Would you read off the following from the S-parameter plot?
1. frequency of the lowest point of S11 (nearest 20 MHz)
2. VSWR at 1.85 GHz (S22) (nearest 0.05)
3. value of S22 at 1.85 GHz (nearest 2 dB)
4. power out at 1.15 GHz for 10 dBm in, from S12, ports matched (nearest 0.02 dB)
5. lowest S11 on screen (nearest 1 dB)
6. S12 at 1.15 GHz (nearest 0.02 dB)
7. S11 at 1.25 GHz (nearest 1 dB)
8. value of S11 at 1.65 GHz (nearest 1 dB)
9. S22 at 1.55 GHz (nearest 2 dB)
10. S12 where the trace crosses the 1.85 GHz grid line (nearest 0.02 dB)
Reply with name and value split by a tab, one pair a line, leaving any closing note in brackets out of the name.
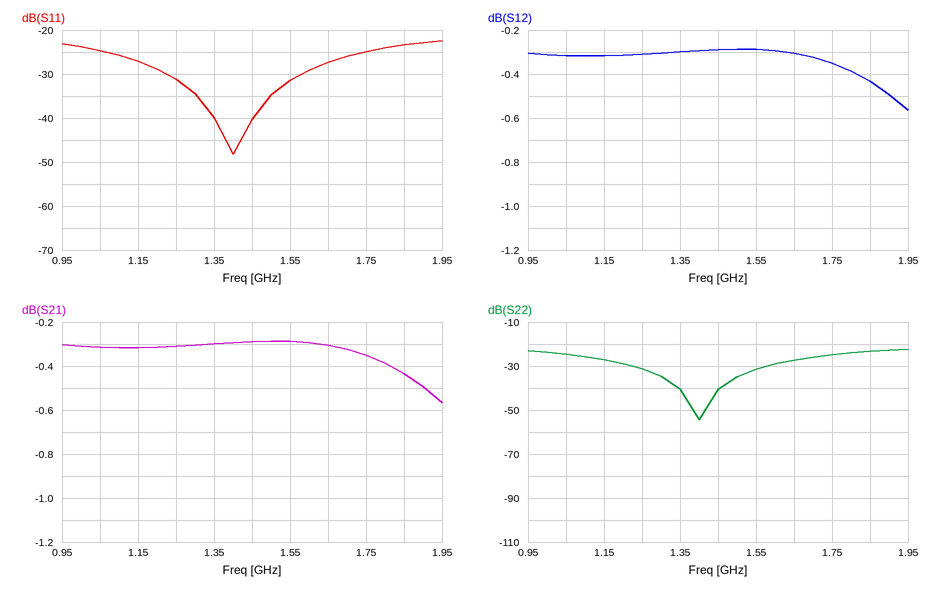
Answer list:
frequency of the lowest point of S11	1.40 GHz
VSWR at 1.85 GHz (S22)	1.15
value of S22 at 1.85 GHz	-24 dB
power out at 1.15 GHz for 10 dBm in, from S12, ports matched	9.68 dBm
lowest S11 on screen	-48 dB
S12 at 1.15 GHz	-0.32 dB
S11 at 1.25 GHz	-31 dB
value of S11 at 1.65 GHz	-27 dB
S22 at 1.55 GHz	-32 dB
S12 where the trace crosses the 1.85 GHz grid line	-0.44 dB
